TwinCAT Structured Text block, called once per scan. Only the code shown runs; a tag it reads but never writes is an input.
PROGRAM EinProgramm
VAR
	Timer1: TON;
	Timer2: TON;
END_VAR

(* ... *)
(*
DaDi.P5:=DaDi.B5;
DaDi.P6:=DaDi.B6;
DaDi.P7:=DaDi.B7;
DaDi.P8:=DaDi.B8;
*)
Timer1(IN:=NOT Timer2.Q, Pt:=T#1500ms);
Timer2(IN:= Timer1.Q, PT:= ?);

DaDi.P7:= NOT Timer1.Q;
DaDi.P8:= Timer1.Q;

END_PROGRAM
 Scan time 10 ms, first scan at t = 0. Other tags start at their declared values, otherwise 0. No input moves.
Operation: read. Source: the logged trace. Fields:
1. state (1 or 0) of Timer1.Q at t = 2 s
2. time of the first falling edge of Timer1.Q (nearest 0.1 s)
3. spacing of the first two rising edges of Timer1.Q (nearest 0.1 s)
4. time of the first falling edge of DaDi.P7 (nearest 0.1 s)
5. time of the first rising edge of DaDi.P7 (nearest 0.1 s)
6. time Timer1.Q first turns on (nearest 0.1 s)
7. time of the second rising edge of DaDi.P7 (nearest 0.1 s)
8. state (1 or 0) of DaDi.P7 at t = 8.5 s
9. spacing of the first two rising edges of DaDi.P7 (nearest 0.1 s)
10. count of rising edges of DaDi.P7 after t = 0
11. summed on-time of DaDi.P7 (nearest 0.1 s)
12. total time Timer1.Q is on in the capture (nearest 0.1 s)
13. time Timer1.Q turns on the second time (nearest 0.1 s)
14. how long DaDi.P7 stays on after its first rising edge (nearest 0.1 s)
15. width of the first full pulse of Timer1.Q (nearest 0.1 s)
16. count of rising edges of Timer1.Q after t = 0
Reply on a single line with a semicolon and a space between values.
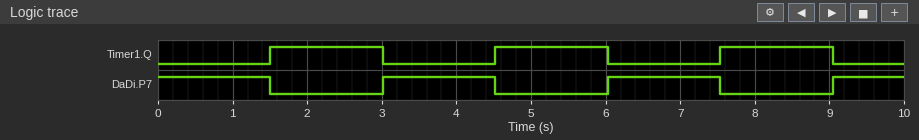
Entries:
1; 3.0 s; 3.0 s; 1.5 s; 3.0 s; 1.5 s; 6.0 s; 0; 3.0 s; 3; 5.5 s; 4.5 s; 4.5 s; 1.5 s; 1.5 s; 3
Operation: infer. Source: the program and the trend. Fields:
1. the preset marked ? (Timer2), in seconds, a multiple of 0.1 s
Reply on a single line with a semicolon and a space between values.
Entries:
1.5 s
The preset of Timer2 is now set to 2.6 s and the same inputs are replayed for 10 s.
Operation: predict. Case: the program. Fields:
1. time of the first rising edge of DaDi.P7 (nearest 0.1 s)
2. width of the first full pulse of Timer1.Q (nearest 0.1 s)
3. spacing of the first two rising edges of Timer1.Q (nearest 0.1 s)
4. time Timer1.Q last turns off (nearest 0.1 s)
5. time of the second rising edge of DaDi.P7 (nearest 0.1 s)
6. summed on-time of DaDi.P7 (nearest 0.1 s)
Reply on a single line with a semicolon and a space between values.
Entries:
4.1 s; 2.6 s; 4.1 s; 8.2 s; 8.2 s; 4.5 s
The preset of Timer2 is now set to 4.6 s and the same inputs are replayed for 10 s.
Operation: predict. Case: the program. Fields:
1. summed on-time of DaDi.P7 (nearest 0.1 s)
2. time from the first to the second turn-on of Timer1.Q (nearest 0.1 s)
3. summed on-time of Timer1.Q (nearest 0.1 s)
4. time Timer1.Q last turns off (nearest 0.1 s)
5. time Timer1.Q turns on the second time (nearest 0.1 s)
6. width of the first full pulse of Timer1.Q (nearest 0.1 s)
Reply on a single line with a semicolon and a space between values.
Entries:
3.0 s; 6.1 s; 7.0 s; 6.1 s; 7.6 s; 4.6 s
